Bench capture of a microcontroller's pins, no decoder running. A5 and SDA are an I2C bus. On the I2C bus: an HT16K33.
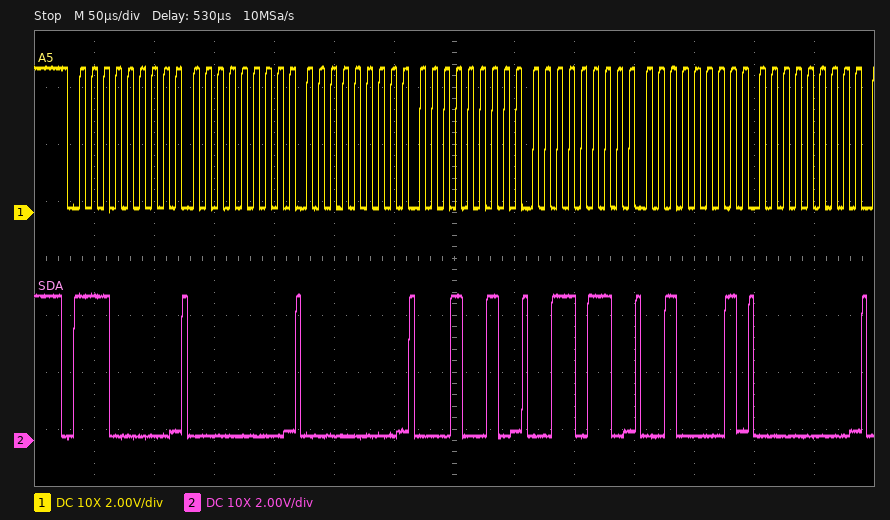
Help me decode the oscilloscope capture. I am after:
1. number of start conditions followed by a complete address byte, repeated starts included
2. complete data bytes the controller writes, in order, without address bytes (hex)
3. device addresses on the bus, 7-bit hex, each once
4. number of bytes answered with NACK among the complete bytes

1
00 00 12 36 21 00
0x70
0
